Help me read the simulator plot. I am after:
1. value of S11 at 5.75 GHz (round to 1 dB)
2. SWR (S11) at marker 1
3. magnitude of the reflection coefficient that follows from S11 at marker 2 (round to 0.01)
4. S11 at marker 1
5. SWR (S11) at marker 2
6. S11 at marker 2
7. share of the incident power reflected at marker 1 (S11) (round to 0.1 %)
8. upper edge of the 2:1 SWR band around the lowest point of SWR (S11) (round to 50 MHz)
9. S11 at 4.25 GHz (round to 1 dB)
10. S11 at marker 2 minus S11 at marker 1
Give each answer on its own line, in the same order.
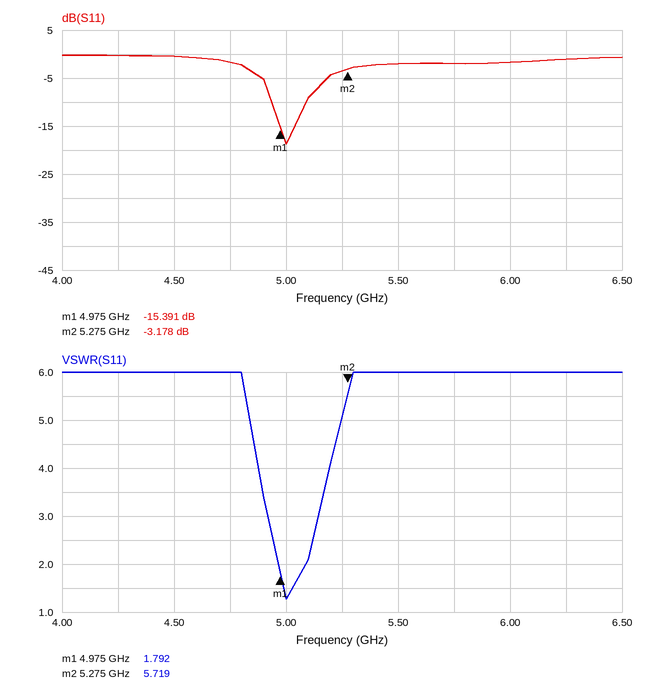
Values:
-2 dB
1.792
0.69
-15.391 dB
5.719
-3.178 dB
2.9 %
5.10 GHz
0 dB
12.213 dB
